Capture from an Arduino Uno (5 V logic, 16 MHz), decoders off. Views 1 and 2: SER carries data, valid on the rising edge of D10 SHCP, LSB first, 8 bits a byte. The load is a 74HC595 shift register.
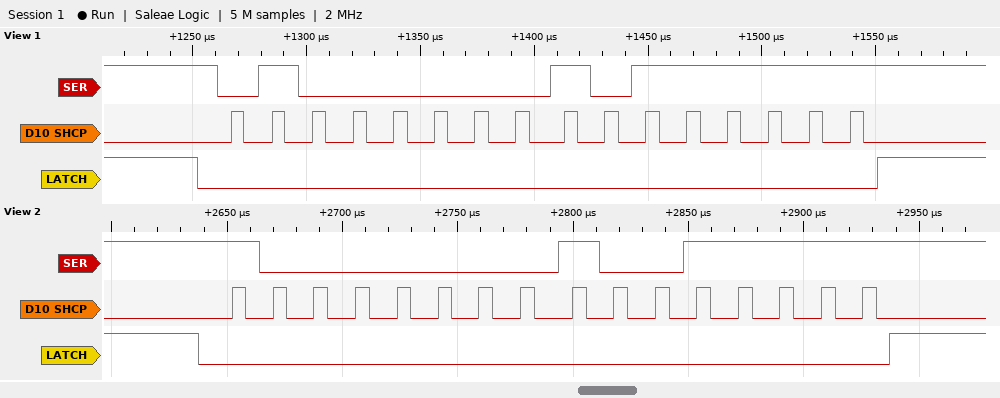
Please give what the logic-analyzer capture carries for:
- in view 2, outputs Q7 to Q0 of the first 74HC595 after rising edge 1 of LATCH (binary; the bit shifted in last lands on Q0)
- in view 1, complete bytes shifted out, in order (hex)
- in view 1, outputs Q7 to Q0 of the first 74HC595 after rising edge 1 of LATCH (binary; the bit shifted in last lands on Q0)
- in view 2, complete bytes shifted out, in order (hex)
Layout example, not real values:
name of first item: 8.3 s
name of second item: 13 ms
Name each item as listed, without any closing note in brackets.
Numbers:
in view 2, outputs Q7 to Q0 of the first 74HC595 after rising edge 1 of LATCH: 10011111
in view 1, complete bytes shifted out, in order: 0x02 0xFD
in view 1, outputs Q7 to Q0 of the first 74HC595 after rising edge 1 of LATCH: 10111111
in view 2, complete bytes shifted out, in order: 0x01 0xF9
